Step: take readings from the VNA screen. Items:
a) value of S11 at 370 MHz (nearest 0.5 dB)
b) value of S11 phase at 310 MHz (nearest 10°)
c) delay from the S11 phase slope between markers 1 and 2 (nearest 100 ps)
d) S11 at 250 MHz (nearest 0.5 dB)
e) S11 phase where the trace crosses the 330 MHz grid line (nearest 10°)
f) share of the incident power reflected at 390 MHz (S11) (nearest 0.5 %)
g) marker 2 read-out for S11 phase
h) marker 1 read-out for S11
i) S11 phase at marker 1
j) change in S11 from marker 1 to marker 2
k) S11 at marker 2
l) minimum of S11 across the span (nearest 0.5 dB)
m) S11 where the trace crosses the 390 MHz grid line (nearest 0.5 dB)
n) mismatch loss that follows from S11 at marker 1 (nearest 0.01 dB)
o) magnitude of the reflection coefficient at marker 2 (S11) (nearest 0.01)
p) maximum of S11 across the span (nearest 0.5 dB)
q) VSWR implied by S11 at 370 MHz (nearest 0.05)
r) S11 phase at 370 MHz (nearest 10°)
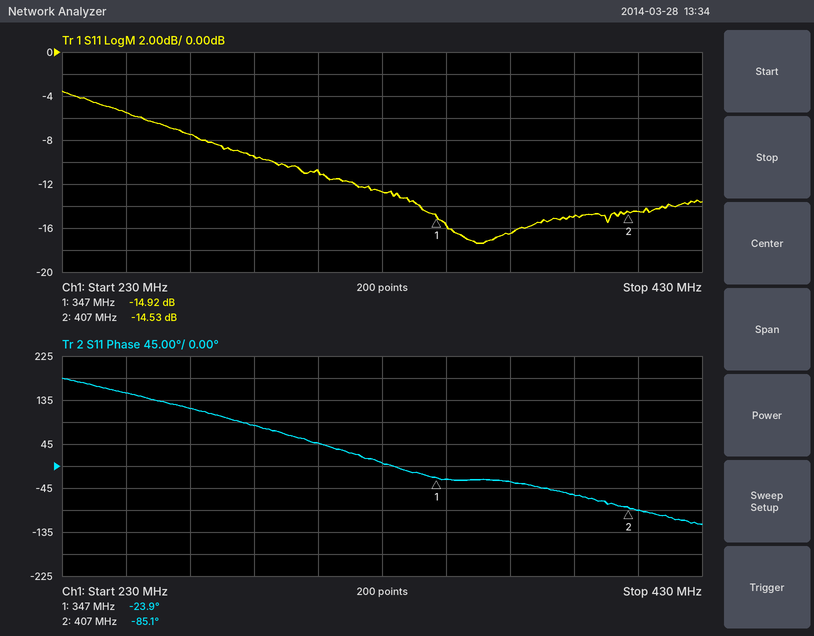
-16.5 dB
50°
2.8 ns
-5.5 dB
10°
3.0 %
-85.1°
-14.92 dB
-23.9°
0.39 dB
-14.53 dB
-17.5 dB
-15.0 dB
0.14 dB
0.19
-3.5 dB
1.35
-30°
